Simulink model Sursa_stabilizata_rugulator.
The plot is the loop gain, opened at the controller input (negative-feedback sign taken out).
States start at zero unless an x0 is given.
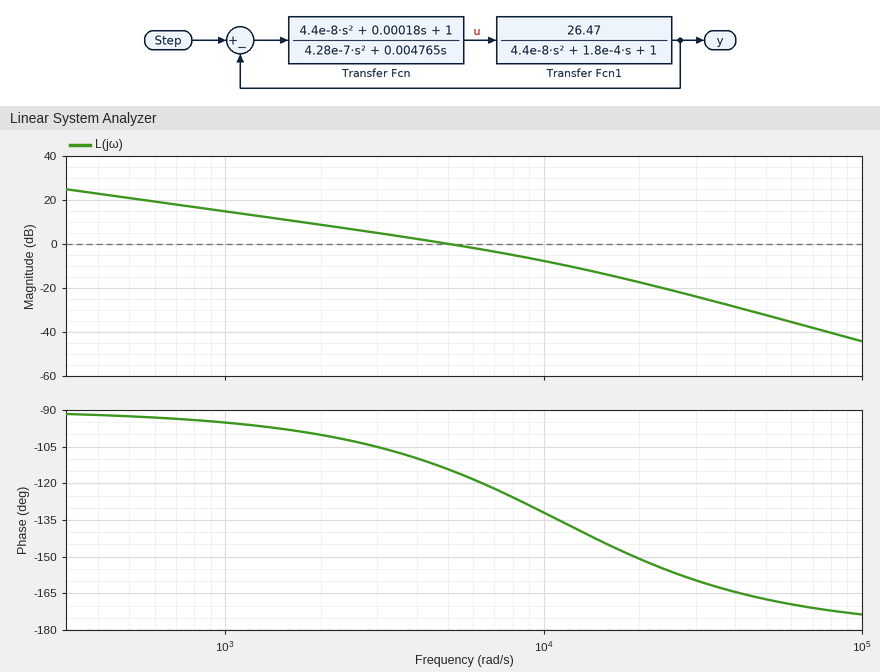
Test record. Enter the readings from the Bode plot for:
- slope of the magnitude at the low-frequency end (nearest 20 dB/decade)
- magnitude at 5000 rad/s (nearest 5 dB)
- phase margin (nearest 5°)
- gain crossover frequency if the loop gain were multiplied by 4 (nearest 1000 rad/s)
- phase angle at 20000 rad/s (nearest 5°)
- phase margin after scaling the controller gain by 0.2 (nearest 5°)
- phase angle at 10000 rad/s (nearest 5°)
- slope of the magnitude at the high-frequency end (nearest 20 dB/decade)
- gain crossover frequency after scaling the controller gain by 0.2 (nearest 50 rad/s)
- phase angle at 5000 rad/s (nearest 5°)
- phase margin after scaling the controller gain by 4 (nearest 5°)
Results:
-20 dB/decade
0 dB
65°
14000 rad/s
-150°
85°
-130°
-40 dB/decade
1100 rad/s
-115°
40°
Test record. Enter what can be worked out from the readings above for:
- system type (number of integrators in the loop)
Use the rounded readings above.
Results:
1
